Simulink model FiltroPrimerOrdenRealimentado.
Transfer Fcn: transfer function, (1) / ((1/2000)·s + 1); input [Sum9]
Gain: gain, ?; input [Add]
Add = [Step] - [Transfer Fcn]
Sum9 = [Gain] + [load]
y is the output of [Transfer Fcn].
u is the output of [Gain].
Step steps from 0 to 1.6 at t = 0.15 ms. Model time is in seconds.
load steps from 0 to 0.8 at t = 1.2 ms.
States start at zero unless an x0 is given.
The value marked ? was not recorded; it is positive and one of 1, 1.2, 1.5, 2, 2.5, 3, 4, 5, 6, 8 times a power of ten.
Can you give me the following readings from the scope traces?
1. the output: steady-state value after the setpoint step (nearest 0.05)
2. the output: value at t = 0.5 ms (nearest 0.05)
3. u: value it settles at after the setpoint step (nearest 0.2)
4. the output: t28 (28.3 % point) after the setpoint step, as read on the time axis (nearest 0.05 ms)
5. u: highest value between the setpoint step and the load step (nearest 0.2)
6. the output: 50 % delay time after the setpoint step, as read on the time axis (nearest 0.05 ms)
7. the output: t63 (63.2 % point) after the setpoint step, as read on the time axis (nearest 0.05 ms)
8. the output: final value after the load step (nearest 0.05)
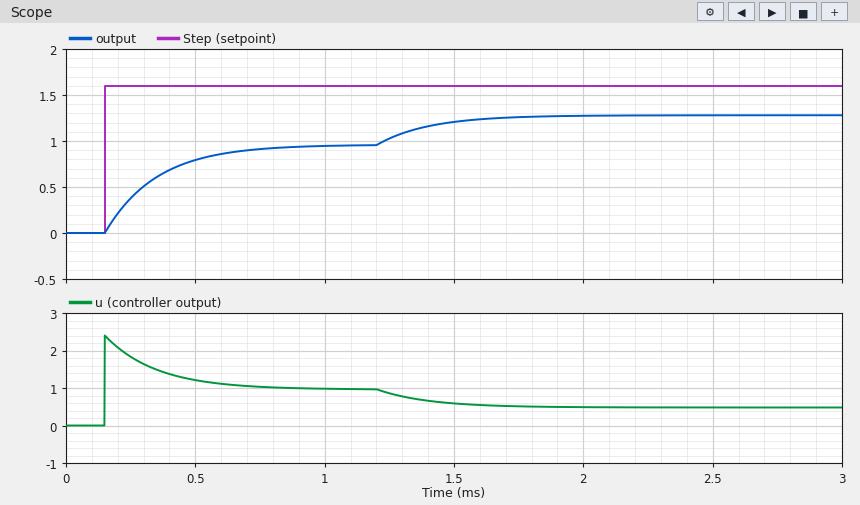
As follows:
0.95
0.80
1.0
0.20 ms
2.4
0.30 ms
0.35 ms
1.30
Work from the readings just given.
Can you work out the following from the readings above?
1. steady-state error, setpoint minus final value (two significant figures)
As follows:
0.65
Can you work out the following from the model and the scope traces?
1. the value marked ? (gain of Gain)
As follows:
1.5
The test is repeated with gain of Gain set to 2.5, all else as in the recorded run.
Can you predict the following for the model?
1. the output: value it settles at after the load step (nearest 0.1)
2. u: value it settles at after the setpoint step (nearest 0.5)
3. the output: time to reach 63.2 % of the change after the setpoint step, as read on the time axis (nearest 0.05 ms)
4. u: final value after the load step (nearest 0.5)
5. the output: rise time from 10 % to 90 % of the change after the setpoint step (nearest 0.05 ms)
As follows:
1.4
1.0
0.30 ms
0.5
0.30 ms
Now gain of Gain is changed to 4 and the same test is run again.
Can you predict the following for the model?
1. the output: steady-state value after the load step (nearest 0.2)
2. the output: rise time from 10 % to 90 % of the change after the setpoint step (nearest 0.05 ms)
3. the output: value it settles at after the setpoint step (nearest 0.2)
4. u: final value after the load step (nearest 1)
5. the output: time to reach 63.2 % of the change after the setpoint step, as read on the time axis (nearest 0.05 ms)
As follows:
1.4
0.20 ms
1.2
1
0.25 ms
